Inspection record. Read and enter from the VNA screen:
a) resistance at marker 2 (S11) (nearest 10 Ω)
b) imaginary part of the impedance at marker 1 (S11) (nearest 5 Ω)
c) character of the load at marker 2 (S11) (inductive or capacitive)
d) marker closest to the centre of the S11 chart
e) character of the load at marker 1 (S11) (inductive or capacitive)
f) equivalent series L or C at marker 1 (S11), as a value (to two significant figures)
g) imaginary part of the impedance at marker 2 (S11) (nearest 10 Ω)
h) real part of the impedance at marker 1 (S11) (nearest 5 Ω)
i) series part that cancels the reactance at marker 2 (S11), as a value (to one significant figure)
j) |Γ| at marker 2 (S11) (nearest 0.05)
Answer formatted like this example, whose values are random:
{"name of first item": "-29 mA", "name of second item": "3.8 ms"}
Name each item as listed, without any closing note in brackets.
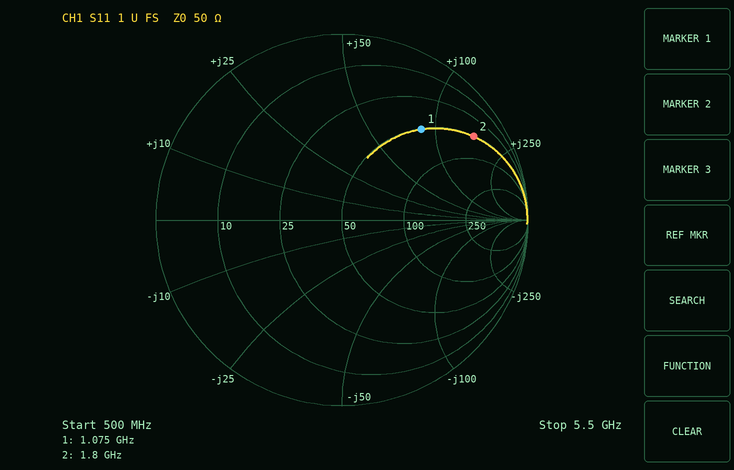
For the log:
{"resistance at marker 2 (S11)": "50 Ω", "imaginary part of the impedance at marker 1 (S11)": "+85 Ω", "character of the load at marker 2 (S11)": "inductive", "marker closest to the centre of the S11 chart": "marker 1", "character of the load at marker 1 (S11)": "inductive", "equivalent series L or C at marker 1 (S11), as a value": "13 nH", "imaginary part of the impedance at marker 2 (S11)": "+160 Ω", "real part of the impedance at marker 1 (S11)": "50 Ω", "series part that cancels the reactance at marker 2 (S11), as a value": "600 fF", "|Γ| at marker 2 (S11)": "0.85"}
